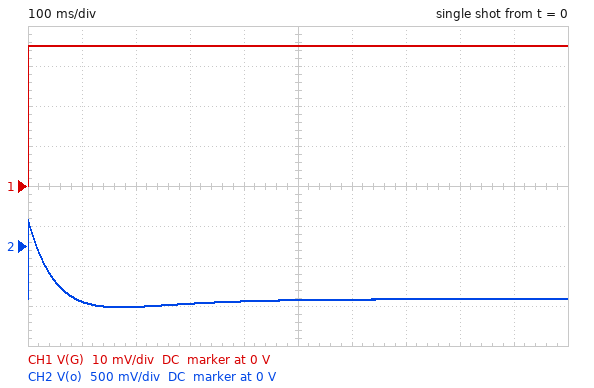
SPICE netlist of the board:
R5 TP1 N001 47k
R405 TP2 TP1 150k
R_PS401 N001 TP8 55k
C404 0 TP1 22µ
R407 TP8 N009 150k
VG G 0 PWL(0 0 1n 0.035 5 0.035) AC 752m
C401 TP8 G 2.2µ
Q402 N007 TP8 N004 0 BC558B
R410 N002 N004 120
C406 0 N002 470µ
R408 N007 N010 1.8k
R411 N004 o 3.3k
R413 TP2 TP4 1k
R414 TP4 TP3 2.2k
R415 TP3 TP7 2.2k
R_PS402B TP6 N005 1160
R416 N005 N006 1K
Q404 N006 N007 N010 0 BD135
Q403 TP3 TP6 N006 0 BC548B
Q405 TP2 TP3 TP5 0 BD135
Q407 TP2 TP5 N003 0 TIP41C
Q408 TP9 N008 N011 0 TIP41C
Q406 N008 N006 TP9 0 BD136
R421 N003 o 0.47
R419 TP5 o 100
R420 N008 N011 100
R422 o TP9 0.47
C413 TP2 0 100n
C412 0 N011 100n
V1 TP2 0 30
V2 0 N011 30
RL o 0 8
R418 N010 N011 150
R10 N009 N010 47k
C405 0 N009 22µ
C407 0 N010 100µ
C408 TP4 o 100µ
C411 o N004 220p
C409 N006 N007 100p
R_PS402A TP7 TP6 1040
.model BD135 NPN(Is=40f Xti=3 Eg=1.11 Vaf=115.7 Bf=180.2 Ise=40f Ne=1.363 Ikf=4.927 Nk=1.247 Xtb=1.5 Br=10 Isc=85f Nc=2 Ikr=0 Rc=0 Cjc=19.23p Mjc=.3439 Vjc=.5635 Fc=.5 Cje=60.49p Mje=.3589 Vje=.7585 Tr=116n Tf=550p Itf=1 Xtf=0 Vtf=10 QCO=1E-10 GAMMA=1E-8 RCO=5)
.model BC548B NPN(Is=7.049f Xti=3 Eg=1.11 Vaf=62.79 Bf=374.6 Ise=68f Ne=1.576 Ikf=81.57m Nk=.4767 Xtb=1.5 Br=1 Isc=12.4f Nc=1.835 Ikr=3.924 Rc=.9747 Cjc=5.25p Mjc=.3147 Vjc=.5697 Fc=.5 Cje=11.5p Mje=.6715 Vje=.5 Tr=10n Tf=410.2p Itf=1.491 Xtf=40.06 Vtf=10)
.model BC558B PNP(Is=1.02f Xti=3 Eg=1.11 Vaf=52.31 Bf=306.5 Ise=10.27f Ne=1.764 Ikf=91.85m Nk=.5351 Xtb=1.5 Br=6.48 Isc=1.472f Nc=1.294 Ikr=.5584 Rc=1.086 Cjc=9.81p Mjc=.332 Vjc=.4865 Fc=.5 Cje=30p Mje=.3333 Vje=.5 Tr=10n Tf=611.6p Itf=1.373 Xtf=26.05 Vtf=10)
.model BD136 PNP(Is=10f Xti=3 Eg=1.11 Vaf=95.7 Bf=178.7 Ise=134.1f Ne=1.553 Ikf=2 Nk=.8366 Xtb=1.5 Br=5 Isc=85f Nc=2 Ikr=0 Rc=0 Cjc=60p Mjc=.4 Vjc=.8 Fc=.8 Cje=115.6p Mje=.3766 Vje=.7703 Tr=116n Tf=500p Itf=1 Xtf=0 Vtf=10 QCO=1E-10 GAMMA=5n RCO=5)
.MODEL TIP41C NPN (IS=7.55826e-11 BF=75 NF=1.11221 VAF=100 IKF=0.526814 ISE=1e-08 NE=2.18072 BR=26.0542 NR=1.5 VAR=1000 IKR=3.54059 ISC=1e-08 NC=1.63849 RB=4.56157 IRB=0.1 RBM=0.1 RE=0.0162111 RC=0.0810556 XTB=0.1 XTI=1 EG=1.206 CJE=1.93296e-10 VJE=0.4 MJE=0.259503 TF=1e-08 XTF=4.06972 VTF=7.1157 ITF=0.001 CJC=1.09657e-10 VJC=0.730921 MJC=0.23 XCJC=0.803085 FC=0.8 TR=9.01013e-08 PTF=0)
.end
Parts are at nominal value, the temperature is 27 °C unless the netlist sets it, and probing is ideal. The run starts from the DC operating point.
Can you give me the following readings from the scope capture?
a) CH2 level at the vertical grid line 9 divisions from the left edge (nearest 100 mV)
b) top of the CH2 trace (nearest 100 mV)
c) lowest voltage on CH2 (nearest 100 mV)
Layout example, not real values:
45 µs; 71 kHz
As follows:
-700 mV; 300 mV; -800 mV
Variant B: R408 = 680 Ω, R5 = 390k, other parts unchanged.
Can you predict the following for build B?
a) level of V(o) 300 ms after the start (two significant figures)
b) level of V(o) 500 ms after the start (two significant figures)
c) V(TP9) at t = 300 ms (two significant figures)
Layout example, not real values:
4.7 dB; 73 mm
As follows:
-9.0 V; -8.9 V; -9.5 V
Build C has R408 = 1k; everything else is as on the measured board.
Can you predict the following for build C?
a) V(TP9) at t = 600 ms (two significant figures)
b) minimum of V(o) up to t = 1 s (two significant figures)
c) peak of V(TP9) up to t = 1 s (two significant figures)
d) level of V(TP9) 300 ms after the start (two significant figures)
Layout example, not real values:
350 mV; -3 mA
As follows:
380 mV; 290 mV; 1.4 V; 330 mV
